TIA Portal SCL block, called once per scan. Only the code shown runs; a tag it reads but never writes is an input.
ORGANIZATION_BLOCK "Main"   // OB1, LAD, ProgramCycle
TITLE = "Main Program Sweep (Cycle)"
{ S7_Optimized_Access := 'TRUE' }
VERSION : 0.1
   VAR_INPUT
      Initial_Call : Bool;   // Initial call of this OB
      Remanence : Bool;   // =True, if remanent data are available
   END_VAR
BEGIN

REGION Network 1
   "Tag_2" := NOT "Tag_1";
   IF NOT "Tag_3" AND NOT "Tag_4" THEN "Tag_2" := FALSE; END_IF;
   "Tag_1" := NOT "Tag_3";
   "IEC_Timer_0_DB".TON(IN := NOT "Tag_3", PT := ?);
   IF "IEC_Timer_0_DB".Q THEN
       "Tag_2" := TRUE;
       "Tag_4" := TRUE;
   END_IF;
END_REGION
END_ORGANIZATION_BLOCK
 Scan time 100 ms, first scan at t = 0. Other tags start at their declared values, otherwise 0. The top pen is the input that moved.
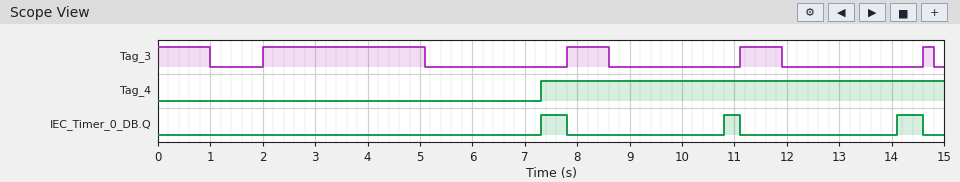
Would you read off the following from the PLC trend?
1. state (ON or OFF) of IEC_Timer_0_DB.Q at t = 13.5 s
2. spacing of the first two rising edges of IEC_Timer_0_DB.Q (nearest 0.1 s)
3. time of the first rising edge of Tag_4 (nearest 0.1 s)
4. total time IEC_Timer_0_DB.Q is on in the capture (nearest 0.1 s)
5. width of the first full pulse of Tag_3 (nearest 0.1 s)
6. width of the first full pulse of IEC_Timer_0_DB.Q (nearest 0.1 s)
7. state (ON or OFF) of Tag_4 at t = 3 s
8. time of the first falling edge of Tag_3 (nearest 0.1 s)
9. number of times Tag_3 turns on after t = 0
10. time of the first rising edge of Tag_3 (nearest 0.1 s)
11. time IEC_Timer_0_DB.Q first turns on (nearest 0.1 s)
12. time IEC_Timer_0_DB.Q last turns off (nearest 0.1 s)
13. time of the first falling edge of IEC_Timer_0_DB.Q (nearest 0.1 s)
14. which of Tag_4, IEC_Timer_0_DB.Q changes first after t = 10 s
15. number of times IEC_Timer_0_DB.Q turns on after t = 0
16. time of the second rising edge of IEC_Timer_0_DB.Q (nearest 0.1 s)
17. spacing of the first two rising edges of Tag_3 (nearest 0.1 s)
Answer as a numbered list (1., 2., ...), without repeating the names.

1. OFF
2. 3.5 s
3. 7.3 s
4. 1.3 s
5. 3.1 s
6. 0.5 s
7. OFF
8. 1.0 s
9. 4
10. 2.0 s
11. 7.3 s
12. 14.6 s
13. 7.8 s
14. IEC_Timer_0_DB.Q
15. 3
16. 10.8 s
17. 5.8 s
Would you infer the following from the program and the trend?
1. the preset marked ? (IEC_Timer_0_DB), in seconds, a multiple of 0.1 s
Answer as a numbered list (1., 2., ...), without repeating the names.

1. 2.2 s
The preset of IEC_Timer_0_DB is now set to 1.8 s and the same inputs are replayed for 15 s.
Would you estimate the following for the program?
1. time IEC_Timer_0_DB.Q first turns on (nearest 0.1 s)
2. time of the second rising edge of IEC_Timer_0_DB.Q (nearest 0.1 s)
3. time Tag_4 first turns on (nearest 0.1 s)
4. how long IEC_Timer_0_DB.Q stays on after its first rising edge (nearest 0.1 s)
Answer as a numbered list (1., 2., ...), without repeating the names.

1. 6.9 s
2. 10.4 s
3. 6.9 s
4. 0.9 s
